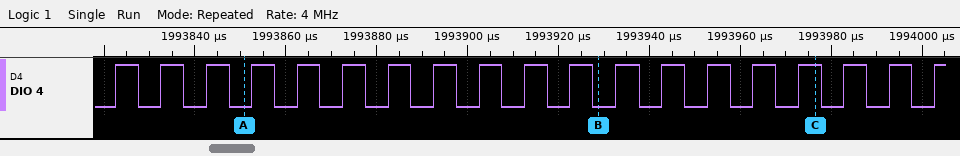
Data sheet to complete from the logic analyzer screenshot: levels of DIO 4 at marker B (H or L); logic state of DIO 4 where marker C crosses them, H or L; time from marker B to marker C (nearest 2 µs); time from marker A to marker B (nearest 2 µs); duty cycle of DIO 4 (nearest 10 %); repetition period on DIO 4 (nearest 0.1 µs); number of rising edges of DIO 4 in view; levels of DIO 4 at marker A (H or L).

DIO 4=L
DIO 4=H
48 µs
78 µs
50 %
10 µs
19
DIO 4=L
